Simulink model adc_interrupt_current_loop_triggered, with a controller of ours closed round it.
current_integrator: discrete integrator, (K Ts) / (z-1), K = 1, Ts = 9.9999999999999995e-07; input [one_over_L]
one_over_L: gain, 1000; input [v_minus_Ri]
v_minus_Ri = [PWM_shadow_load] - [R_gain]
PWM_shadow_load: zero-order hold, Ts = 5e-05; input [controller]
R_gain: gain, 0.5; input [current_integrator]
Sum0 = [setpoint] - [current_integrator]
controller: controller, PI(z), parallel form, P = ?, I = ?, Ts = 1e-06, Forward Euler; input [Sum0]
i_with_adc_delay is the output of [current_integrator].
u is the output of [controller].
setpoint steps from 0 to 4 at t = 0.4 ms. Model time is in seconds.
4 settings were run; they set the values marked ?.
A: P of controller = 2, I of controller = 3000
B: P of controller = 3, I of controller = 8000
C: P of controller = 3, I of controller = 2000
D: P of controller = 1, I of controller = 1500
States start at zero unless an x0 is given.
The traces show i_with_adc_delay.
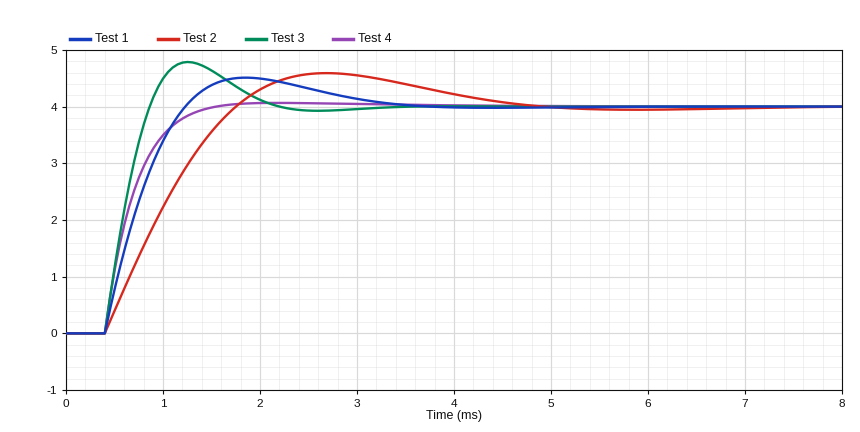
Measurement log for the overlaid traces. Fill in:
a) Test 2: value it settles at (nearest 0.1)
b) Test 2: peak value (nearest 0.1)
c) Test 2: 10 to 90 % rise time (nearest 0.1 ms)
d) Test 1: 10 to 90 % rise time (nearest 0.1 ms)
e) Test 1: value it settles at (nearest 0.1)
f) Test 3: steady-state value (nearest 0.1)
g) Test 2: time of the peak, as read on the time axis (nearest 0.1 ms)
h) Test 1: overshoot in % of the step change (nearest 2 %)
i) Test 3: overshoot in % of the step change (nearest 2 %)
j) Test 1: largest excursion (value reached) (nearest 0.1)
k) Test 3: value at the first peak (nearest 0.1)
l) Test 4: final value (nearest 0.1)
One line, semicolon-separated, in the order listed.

4.0; 4.6; 1.0 ms; 0.6 ms; 4.0; 4.0; 2.7 ms; 12 %; 20 %; 4.5; 4.8; 4.0
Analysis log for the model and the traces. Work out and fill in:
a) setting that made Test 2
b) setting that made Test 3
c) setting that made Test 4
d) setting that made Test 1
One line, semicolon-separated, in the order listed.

D; B; C; A
